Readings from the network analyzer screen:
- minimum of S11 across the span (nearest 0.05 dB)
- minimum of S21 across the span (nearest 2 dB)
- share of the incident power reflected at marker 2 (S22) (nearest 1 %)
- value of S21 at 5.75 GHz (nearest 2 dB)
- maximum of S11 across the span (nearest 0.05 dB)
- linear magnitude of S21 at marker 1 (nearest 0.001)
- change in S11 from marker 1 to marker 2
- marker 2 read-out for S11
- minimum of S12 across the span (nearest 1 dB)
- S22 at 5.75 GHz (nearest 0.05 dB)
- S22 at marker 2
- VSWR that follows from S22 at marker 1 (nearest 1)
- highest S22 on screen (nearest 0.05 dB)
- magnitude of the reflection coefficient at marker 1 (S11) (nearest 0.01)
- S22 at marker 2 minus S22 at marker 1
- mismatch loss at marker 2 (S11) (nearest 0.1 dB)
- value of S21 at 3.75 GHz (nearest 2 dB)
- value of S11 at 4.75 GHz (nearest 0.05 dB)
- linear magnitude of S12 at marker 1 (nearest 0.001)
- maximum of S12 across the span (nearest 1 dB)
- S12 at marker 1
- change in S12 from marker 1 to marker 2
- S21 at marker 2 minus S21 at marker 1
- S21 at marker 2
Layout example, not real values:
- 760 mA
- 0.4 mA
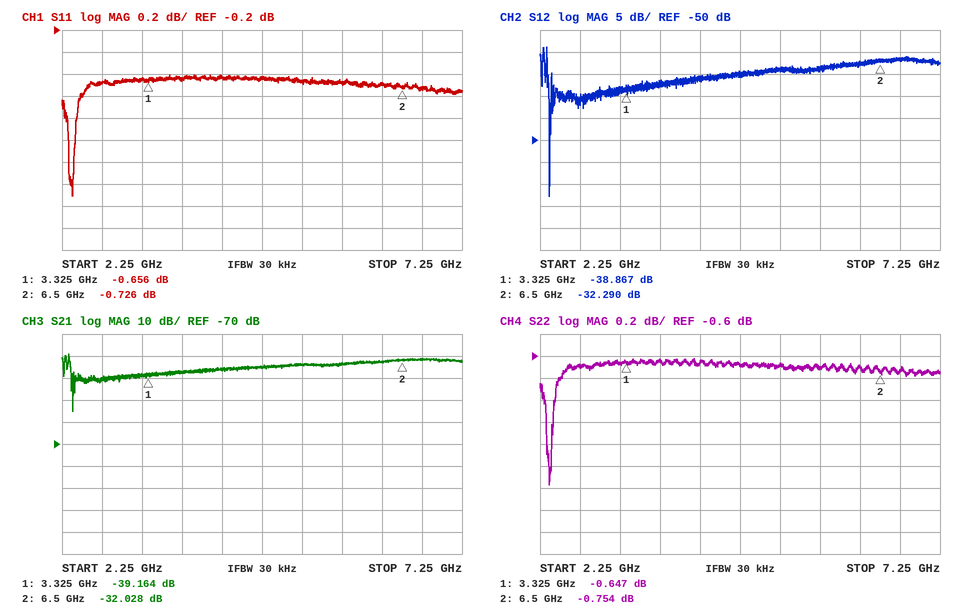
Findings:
- -1.70 dB
- -56 dB
- 84 %
- -34 dB
- -0.60 dB
- 0.011
- -0.070 dB
- -0.726 dB
- -63 dB
- -0.70 dB
- -0.754 dB
- 27
- -0.60 dB
- 0.93
- -0.107 dB
- 8.1 dB
- -38 dB
- -0.65 dB
- 0.011
- -29 dB
- -38.867 dB
- 6.577 dB
- 7.136 dB
- -32.028 dB
